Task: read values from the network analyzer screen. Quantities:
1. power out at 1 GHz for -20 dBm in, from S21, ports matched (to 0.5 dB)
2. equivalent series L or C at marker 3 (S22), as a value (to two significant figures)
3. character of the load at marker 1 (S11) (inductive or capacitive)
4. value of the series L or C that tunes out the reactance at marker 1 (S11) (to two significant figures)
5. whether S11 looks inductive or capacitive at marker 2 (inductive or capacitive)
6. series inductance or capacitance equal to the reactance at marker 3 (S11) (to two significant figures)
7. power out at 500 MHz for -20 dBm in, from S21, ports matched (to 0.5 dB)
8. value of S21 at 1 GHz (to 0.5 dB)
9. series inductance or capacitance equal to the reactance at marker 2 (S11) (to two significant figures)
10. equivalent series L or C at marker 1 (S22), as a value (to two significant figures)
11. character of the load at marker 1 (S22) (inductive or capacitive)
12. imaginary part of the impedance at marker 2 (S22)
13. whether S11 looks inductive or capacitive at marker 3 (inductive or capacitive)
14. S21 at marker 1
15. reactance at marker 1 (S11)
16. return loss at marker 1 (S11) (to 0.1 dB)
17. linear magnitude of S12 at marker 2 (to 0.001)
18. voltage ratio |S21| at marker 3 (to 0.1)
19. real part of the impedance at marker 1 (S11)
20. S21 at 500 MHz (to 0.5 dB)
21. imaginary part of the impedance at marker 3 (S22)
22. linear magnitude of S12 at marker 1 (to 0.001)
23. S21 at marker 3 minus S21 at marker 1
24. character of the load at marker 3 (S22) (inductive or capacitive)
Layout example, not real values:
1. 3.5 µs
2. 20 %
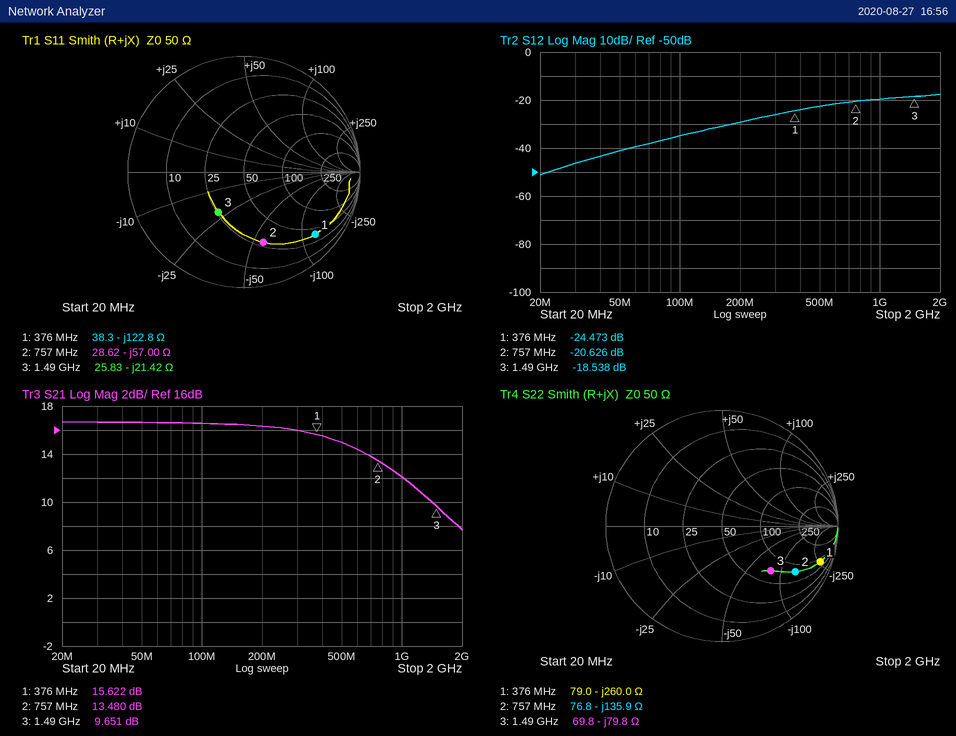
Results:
1. -8.0 dBm
2. 1.3 pF
3. capacitive
4. 52 nH
5. capacitive
6. 5.0 pF
7. -5.0 dBm
8. 12.0 dB
9. 3.7 pF
10. 1.6 pF
11. capacitive
12. -135.9 Ω
13. capacitive
14. 15.622 dB
15. -122.8 Ω
16. 1.8 dB
17. 0.093
18. 3.0
19. 38.3 Ω
20. 15.0 dB
21. -79.8 Ω
22. 0.060
23. -5.971 dB
24. capacitive
